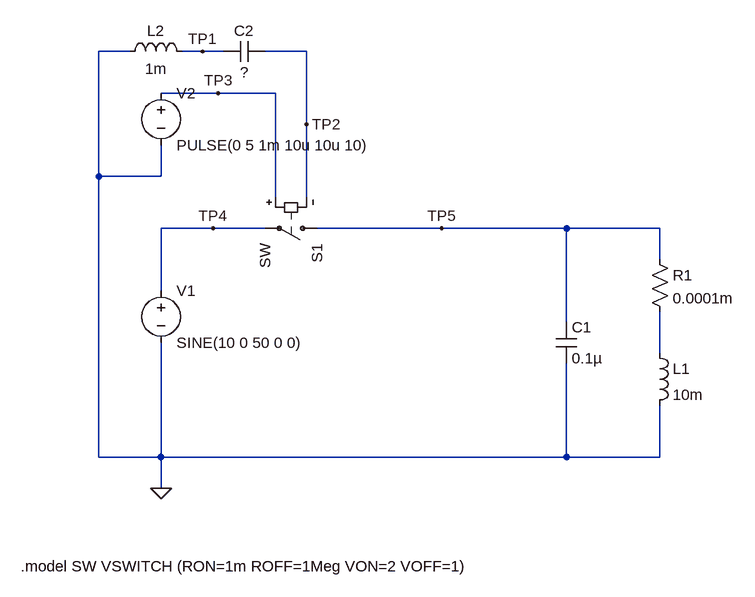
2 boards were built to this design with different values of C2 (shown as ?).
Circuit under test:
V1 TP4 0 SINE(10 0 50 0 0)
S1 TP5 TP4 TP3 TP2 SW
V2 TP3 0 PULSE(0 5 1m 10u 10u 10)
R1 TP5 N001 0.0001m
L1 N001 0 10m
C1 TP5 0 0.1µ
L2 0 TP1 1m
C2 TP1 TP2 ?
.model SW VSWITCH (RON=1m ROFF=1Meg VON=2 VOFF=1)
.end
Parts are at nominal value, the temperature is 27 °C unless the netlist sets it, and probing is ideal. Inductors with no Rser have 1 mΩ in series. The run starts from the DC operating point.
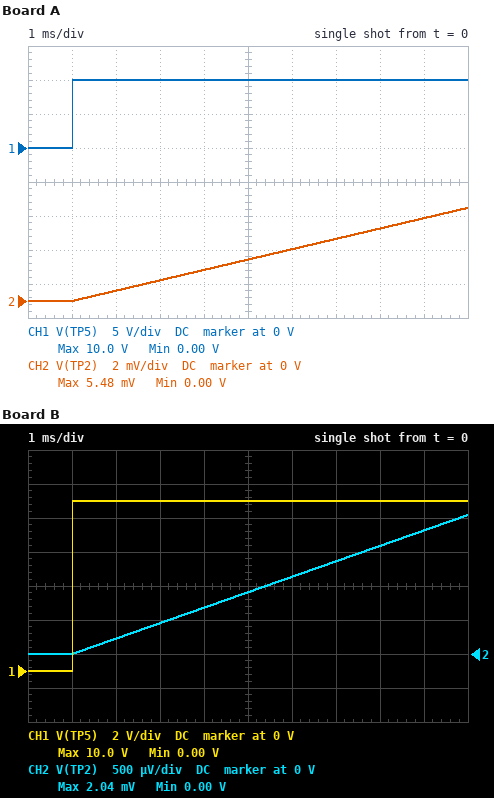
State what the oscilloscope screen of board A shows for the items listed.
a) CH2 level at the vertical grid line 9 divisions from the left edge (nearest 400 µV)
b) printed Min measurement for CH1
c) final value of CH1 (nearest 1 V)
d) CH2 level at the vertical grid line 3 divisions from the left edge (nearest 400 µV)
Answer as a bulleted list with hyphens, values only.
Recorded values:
- 4.8 mV
- 0.00 V
- 10 V
- 1.2 mV
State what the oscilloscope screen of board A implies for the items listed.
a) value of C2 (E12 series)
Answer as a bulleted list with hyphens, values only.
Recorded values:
- 8.2 pF
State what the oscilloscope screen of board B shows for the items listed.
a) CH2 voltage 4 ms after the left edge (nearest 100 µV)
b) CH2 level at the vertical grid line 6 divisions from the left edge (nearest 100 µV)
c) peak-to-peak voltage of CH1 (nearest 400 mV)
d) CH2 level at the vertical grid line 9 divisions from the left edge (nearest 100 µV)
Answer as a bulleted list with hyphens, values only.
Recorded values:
- 700 µV
- 1.1 mV
- 10.0 V
- 1.8 mV
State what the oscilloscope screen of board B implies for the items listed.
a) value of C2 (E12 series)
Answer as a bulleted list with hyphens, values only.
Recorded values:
- 22 pF
